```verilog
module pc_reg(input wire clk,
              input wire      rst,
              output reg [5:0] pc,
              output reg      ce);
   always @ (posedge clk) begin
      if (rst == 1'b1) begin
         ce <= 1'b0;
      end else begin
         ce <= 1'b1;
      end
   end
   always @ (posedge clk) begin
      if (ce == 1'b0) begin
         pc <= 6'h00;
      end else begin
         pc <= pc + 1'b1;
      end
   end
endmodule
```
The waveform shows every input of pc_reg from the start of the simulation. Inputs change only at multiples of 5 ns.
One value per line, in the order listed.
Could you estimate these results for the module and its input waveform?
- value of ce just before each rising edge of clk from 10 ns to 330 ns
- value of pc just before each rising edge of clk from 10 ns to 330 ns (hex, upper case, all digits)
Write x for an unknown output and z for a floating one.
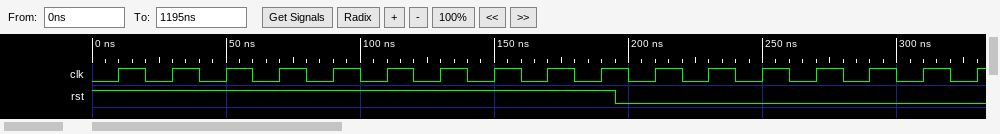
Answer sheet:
x 0 0 0 0 0 0 0 0 0 0 1 1 1 1 1 1
x, x, 00, 00, 00, 00, 00, 00, 00, 00, 00, 00, 01, 02, 03, 04, 05
